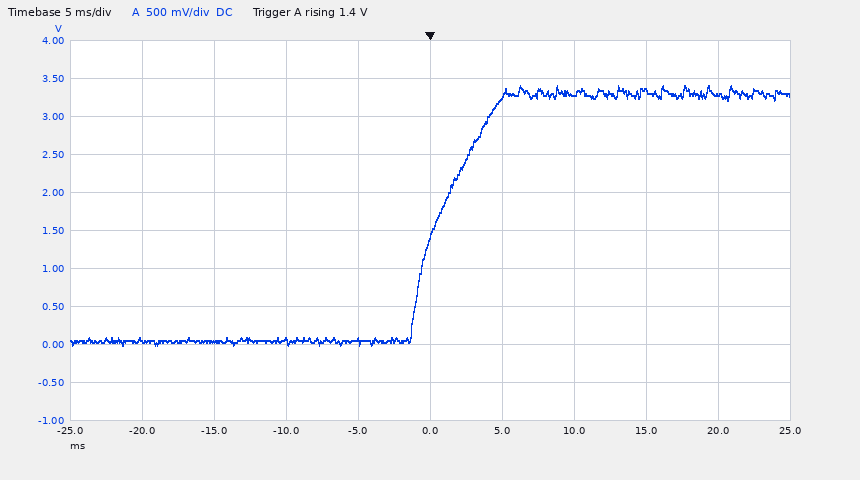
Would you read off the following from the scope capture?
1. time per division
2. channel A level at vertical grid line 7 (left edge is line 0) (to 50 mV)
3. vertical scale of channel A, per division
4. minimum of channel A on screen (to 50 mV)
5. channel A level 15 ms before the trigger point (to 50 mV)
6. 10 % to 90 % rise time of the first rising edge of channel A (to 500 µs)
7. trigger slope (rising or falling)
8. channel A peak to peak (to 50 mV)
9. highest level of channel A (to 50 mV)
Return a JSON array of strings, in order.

["5 ms", "3.30 V", "500 mV", "0 mV", "50 mV", "5.0 ms", "rising", "3.40 V", "3.40 V"]
